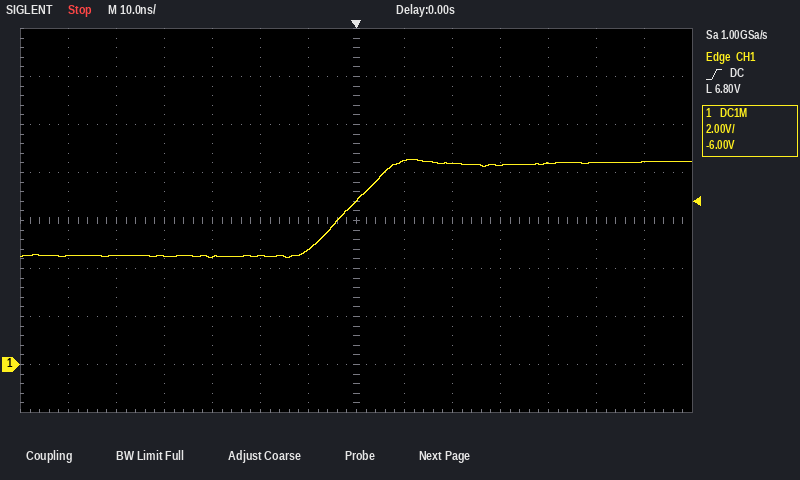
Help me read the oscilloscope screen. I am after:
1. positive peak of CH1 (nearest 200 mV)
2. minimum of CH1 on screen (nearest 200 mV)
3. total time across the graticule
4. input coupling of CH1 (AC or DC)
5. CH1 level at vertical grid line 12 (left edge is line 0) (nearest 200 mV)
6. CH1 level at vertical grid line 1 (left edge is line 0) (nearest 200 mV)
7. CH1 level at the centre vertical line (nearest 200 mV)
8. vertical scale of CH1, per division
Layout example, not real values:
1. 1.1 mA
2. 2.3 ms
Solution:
1. 8.6 V
2. 4.4 V
3. 140 ns
4. DC
5. 8.4 V
6. 4.6 V
7. 6.8 V
8. 2 V
